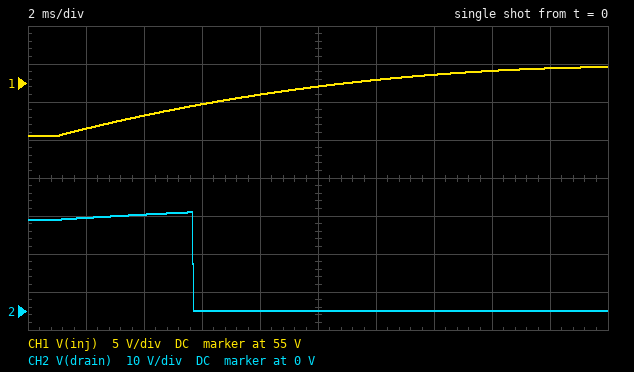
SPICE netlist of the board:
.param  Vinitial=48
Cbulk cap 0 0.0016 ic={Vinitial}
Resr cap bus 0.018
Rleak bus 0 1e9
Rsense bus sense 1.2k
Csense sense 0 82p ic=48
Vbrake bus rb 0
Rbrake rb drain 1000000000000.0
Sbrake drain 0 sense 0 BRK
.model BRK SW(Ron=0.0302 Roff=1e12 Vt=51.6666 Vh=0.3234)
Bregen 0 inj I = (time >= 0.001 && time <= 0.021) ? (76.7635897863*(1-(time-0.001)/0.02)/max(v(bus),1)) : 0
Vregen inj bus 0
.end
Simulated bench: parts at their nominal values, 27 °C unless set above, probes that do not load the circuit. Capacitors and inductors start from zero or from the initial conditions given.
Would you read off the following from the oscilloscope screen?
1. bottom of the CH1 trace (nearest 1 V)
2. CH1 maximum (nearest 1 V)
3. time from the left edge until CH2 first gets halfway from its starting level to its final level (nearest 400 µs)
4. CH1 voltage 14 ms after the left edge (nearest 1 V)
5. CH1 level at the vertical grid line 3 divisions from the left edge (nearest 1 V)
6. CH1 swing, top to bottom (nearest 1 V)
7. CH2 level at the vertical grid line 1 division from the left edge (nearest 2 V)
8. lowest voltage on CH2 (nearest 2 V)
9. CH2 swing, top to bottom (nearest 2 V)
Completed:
48 V
57 V
5.6 ms
56 V
52 V
9 V
24 V
0 V
26 V
